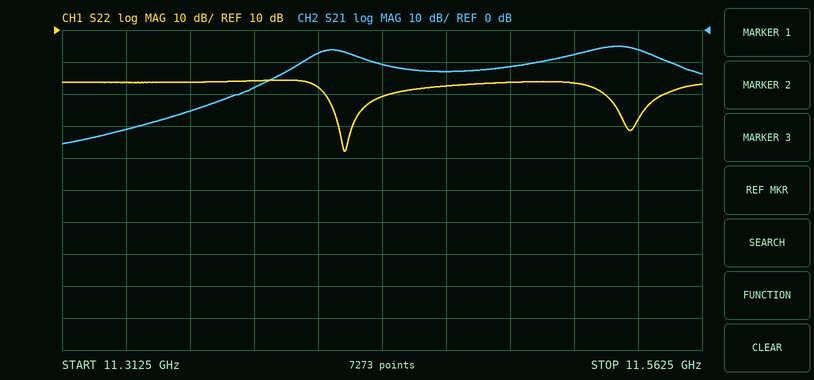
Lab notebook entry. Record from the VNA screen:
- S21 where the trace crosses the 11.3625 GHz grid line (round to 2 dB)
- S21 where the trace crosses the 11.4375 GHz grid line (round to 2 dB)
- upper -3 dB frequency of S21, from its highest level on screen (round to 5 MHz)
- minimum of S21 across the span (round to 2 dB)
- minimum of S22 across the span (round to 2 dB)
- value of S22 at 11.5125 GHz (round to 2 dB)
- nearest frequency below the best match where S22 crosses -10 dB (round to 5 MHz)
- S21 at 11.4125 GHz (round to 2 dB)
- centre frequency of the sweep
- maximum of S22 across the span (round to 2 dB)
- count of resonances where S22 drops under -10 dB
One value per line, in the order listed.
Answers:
-26 dB
-10 dB
11.545 GHz
-36 dB
-28 dB
-6 dB
11.415 GHz
-8 dB
11.4375 GHz
-6 dB
2
